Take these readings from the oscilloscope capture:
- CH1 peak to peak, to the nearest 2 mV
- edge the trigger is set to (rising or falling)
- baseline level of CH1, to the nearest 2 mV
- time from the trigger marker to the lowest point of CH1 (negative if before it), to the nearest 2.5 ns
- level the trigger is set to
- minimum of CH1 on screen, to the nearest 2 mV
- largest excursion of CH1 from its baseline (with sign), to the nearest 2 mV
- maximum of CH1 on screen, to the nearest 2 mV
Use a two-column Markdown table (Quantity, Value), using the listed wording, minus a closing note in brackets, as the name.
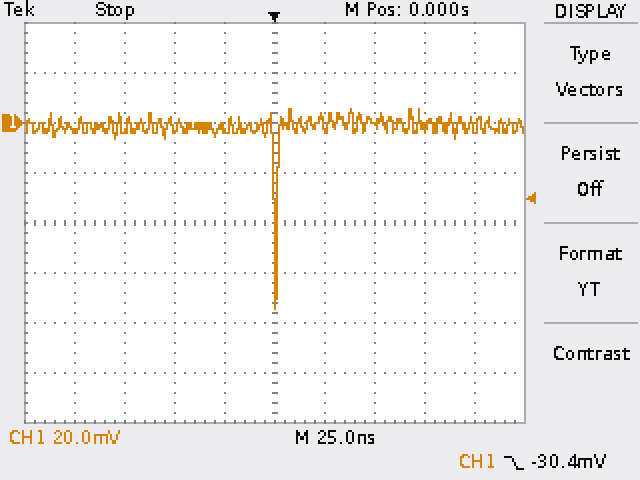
| Quantity | Value |
|---|---|
| CH1 peak to peak, to the nearest 2 mV | 80 mV |
| edge the trigger is set to | falling |
| baseline level of CH1, to the nearest 2 mV | -2 mV |
| time from the trigger marker to the lowest point of CH1 (negative if before it), to the nearest 2.5 ns | 0.0 ns |
| level the trigger is set to | -30.4 mV |
| minimum of CH1 on screen, to the nearest 2 mV | -74 mV |
| largest excursion of CH1 from its baseline (with sign), to the nearest 2 mV | -72 mV |
| maximum of CH1 on screen, to the nearest 2 mV | 6 mV |
